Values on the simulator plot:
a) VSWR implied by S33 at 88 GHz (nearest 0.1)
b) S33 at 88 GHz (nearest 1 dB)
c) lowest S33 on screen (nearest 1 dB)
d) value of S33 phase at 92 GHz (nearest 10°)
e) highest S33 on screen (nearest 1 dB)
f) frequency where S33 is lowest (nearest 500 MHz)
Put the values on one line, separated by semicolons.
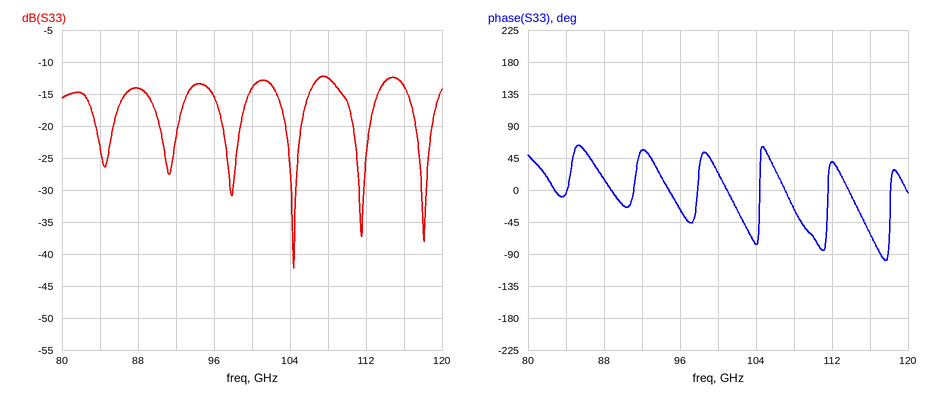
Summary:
1.5; -14 dB; -42 dB; 60°; -12 dB; 104.5 GHz
